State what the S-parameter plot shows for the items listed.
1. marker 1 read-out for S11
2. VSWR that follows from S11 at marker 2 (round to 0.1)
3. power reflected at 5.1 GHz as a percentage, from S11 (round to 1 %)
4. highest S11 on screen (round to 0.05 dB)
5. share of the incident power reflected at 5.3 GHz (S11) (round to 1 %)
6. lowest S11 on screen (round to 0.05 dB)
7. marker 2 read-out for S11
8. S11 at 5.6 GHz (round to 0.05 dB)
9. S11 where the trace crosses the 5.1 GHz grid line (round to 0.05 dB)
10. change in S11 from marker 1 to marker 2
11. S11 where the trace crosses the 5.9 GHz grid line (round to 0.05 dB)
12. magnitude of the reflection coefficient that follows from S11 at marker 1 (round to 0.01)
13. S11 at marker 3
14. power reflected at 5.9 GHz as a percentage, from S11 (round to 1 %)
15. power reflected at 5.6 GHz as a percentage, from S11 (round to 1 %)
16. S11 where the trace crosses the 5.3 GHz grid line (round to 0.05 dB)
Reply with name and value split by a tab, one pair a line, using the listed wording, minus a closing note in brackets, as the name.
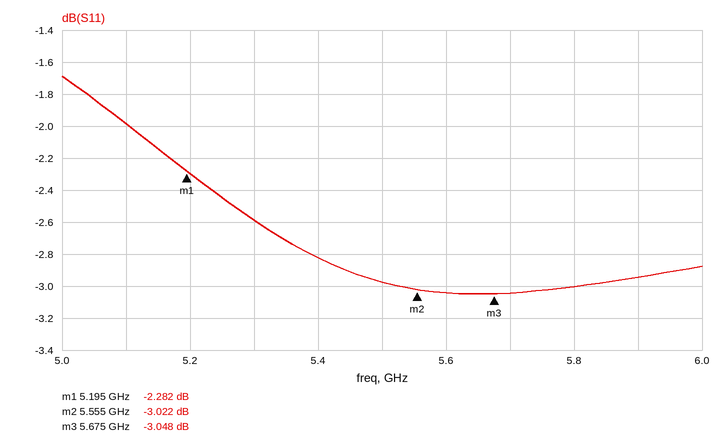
marker 1 read-out for S11	-2.282 dB
VSWR that follows from S11 at marker 2	5.8
power reflected at 5.1 GHz as a percentage, from S11	63 %
highest S11 on screen	-1.70 dB
share of the incident power reflected at 5.3 GHz (S11)	55 %
lowest S11 on screen	-3.05 dB
marker 2 read-out for S11	-3.022 dB
S11 at 5.6 GHz	-3.05 dB
S11 where the trace crosses the 5.1 GHz grid line	-2.00 dB
change in S11 from marker 1 to marker 2	-0.740 dB
S11 where the trace crosses the 5.9 GHz grid line	-2.95 dB
magnitude of the reflection coefficient that follows from S11 at marker 1	0.77
S11 at marker 3	-3.048 dB
power reflected at 5.9 GHz as a percentage, from S11	51 %
power reflected at 5.6 GHz as a percentage, from S11	50 %
S11 where the trace crosses the 5.3 GHz grid line	-2.60 dB
